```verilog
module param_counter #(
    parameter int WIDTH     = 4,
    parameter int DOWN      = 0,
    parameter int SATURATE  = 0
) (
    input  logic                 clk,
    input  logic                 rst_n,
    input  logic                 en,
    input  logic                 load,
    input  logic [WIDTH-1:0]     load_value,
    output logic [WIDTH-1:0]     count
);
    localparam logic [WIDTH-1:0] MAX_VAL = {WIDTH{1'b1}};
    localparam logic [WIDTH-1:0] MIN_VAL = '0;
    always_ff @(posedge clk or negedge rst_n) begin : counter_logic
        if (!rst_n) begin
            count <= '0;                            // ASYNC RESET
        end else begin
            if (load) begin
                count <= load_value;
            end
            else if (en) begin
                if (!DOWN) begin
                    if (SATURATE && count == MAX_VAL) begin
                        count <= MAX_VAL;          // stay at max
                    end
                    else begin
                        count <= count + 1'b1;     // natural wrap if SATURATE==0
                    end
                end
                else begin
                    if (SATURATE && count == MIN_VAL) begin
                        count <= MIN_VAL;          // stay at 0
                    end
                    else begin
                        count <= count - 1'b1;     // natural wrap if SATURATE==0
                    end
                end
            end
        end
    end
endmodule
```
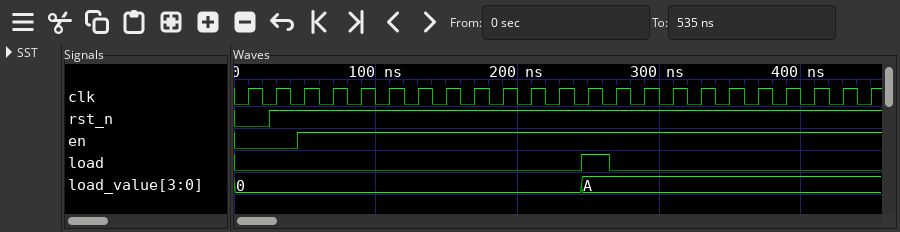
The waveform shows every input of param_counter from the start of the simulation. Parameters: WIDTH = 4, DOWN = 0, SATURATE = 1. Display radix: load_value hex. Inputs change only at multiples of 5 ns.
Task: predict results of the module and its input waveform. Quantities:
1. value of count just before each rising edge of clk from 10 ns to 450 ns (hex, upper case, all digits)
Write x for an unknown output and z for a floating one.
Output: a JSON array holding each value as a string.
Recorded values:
["0, 0, 0, 1, 2, 3, 4, 5, 6, 7, 8, 9, A, A, B, C, D, E, F, F, F, F, F"]
